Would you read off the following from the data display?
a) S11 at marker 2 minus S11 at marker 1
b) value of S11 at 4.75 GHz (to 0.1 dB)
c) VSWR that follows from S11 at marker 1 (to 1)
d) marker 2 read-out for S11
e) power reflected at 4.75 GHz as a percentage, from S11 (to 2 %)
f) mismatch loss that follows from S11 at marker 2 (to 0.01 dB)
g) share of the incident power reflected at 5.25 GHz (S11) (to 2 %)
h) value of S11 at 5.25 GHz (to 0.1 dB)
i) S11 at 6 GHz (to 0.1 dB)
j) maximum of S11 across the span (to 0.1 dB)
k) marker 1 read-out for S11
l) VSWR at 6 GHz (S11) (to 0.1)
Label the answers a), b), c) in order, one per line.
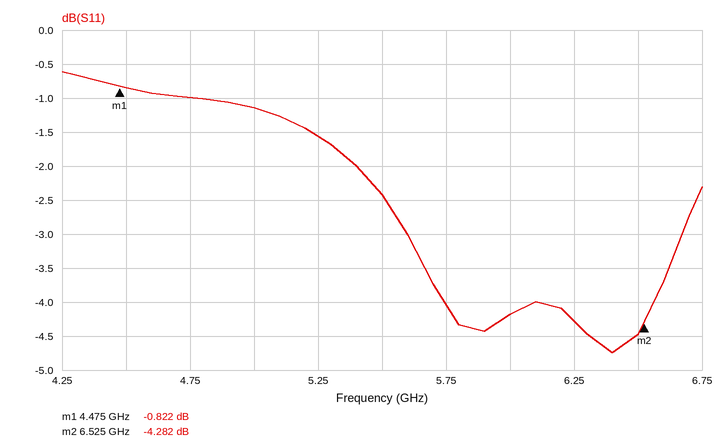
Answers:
a) -3.460 dB
b) -1.0 dB
c) 21
d) -4.282 dB
e) 80 %
f) 2.03 dB
g) 70 %
h) -1.6 dB
i) -4.2 dB
j) -0.6 dB
k) -0.822 dB
l) 4.2
